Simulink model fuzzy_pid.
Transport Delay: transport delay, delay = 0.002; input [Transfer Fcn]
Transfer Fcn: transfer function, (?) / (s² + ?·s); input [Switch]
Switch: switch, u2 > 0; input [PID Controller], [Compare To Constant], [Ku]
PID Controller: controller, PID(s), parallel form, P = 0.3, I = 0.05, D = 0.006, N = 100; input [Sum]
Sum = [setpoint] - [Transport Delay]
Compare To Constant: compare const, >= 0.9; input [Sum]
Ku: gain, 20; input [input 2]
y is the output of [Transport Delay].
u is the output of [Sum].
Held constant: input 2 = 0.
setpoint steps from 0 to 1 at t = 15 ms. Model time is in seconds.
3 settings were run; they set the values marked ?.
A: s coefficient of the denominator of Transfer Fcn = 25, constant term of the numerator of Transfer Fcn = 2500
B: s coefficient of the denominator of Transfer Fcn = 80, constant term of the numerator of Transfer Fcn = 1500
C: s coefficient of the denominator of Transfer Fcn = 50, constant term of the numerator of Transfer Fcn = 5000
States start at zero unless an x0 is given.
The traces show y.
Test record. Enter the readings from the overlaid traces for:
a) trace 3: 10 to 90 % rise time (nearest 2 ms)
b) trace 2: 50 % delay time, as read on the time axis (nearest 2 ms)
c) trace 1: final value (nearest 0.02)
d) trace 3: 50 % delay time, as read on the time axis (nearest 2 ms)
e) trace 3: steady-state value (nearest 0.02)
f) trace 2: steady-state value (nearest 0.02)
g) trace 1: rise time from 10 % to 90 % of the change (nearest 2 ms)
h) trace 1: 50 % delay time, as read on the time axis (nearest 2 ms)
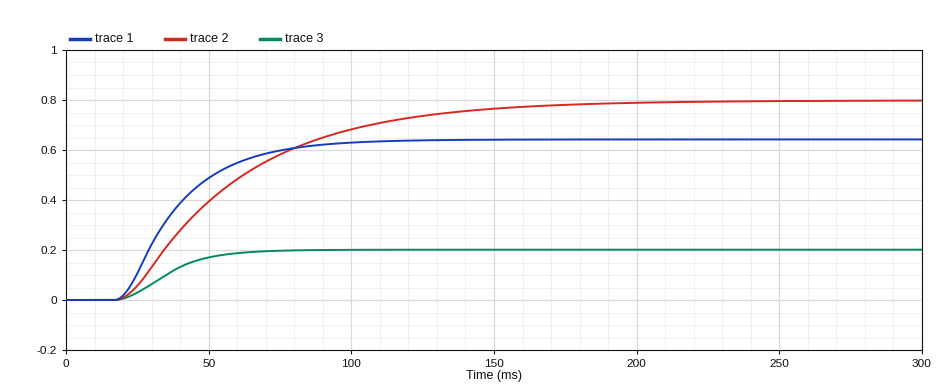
32 ms
50 ms
0.64
36 ms
0.20
0.80
44 ms
36 ms
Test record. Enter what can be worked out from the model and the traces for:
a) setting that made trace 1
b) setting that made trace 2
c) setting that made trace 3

C
A
B
